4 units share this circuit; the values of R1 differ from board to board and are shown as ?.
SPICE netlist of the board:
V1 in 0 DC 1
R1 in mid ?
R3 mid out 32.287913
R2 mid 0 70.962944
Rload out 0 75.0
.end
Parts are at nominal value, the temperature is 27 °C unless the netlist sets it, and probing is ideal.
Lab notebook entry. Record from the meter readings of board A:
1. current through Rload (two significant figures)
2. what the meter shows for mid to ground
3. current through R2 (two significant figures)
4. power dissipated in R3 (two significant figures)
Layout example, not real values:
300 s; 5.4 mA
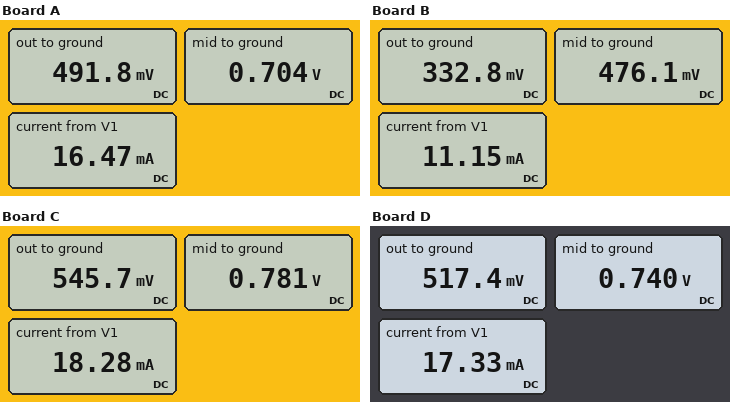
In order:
6.6 mA; 0.704 V; 9.9 mA; 1.4 mW
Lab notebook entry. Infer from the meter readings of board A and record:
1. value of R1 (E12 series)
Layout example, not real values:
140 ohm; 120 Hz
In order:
18 Ω
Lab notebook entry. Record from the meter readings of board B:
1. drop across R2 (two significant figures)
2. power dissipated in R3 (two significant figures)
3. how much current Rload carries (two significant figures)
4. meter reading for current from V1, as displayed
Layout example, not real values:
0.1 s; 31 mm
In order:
480 mV; 640 µW; 4.4 mA; 11.15 mA
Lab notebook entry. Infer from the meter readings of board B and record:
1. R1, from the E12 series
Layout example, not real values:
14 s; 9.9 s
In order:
47 Ω
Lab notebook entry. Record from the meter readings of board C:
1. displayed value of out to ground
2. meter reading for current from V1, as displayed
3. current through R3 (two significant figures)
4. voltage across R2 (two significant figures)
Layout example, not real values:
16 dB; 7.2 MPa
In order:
545.7 mV; 18.28 mA; 7.3 mA; 780 mV
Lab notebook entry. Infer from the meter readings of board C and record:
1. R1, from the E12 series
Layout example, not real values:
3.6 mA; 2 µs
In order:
12 Ω
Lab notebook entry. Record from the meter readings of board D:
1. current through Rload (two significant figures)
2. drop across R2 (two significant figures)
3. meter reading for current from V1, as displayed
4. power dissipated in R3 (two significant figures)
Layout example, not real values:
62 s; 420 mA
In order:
6.9 mA; 740 mV; 17.33 mA; 1.5 mW
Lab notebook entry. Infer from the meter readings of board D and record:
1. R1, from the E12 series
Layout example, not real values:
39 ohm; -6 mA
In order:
15 Ω
